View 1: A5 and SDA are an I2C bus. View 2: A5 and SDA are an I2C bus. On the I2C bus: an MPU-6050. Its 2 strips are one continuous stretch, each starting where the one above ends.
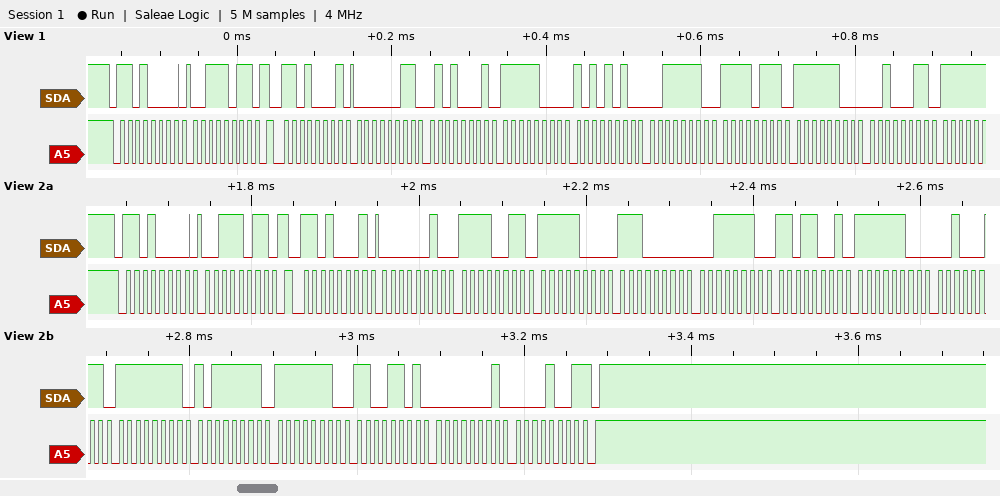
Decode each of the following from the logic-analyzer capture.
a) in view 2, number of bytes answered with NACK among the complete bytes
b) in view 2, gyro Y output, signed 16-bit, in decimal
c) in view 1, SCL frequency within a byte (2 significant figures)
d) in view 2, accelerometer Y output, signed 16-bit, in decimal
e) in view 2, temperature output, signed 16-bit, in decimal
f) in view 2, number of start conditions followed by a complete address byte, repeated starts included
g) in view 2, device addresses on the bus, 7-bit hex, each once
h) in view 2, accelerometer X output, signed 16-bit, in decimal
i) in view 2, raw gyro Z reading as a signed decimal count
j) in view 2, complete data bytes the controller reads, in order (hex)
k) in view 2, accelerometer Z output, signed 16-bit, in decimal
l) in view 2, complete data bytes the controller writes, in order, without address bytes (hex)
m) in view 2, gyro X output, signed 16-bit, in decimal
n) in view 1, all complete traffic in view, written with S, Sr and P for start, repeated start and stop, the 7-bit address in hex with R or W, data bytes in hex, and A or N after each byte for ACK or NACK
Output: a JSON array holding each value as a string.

["1", "-307", "100 kHz", "-1824", "-989", "2", "0x68", "755", "265", "02 F3 F8 E0 3E D9 FC 23 FF BF FE CD 01 09", "16089", "3B", "-65", "S 68W A 3B A Sr 68R A 03 A 51 A F8 A AA A 3E A F7 A FC A 23 A"]
